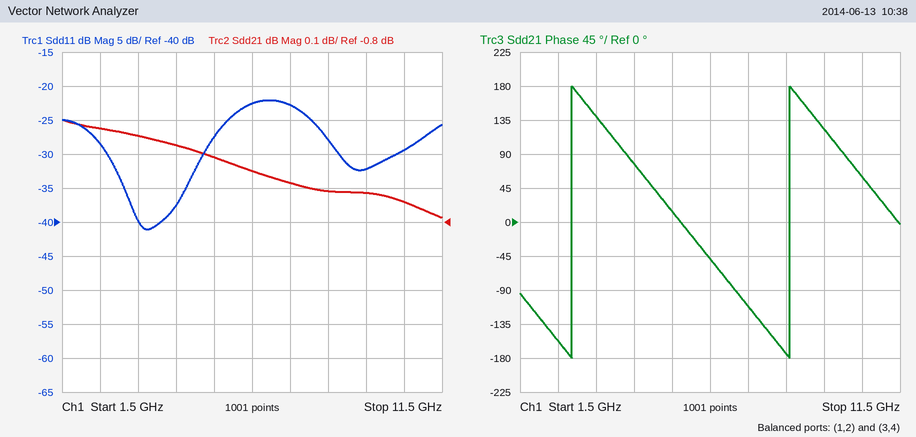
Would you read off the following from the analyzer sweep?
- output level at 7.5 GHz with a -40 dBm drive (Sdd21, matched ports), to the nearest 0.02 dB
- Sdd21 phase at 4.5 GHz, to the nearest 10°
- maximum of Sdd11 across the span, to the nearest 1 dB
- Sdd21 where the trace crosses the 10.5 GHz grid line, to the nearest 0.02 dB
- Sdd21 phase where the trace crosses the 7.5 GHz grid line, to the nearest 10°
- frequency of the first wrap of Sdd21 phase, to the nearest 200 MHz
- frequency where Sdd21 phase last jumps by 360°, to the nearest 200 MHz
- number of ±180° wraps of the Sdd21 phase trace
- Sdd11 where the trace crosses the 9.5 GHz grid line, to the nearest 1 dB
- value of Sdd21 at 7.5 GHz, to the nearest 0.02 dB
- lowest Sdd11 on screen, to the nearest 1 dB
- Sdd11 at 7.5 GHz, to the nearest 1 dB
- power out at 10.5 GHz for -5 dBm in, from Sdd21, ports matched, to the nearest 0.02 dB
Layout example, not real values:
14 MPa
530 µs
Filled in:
-40.68 dBm
80°
-22 dB
-0.74 dB
-110°
2.8 GHz
8.6 GHz
2
-32 dB
-0.68 dB
-41 dB
-23 dB
-5.74 dBm
